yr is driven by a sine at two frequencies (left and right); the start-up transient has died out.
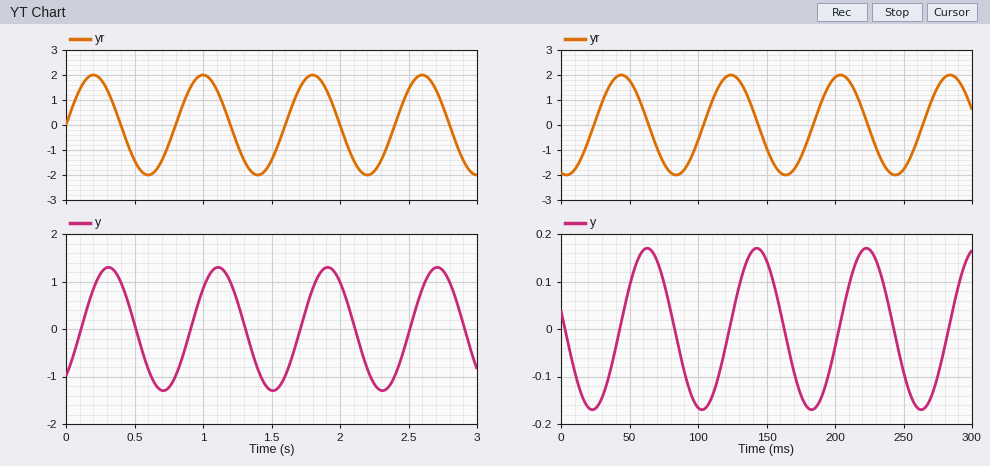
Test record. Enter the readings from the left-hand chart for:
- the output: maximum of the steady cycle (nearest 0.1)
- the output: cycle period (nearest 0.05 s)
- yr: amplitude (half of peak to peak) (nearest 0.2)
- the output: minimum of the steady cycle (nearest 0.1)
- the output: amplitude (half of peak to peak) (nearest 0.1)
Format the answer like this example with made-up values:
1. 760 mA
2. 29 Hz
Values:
1. 1.3
2. 0.80 s
3. 2.0
4. -1.3
5. 1.3
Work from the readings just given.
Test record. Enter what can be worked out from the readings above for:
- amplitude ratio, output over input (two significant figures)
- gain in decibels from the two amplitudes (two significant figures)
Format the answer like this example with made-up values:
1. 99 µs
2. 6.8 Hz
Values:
1. 0.65
2. -3.7 dB
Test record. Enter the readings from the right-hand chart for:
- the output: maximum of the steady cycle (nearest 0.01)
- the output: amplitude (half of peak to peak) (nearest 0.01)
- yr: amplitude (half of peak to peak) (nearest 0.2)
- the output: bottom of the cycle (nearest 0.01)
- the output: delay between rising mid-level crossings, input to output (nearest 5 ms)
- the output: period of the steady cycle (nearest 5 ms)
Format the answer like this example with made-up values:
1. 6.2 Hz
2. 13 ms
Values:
1. 0.17
2. 0.17
3. 2.0
4. -0.17
5. 20 ms
6. 80 ms
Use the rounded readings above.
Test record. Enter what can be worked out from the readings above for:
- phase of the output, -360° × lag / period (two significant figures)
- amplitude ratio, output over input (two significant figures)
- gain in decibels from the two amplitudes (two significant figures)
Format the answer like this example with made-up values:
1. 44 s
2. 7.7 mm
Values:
1. -90°
2. 0.085
3. -21 dB
